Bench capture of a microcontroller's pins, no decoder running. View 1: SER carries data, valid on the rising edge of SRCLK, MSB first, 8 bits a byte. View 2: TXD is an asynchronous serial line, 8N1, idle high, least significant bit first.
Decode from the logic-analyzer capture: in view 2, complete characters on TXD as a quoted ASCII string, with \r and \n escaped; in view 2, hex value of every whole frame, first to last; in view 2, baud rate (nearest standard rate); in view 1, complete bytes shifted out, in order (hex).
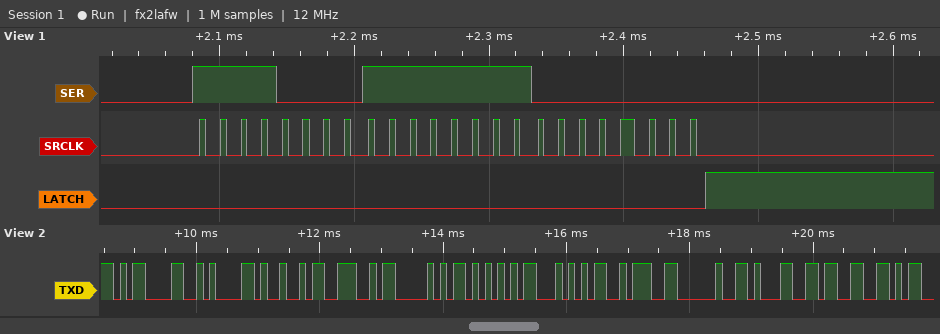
"\r\nINPUT: 13"
0D 0A 49 4E 50 55 54 3A 20 31 33
9600 baud
F0 FF 00
